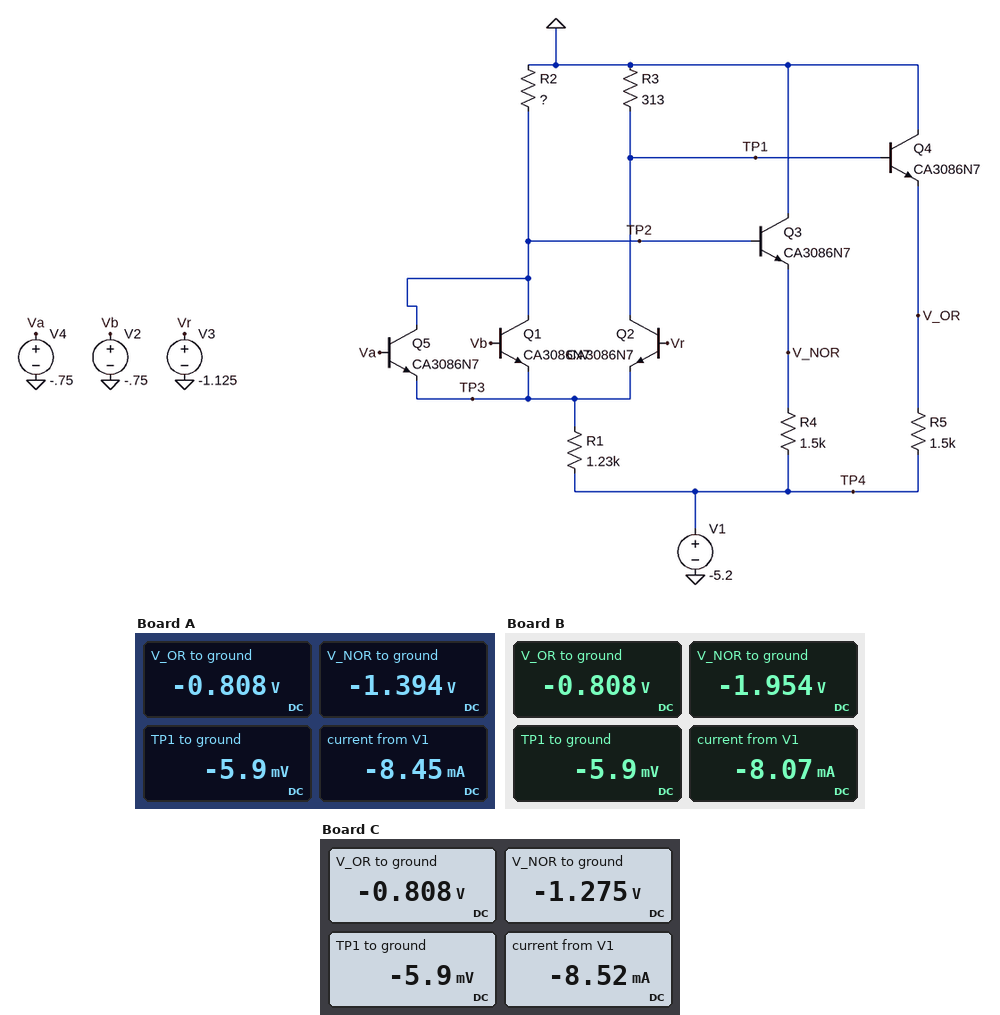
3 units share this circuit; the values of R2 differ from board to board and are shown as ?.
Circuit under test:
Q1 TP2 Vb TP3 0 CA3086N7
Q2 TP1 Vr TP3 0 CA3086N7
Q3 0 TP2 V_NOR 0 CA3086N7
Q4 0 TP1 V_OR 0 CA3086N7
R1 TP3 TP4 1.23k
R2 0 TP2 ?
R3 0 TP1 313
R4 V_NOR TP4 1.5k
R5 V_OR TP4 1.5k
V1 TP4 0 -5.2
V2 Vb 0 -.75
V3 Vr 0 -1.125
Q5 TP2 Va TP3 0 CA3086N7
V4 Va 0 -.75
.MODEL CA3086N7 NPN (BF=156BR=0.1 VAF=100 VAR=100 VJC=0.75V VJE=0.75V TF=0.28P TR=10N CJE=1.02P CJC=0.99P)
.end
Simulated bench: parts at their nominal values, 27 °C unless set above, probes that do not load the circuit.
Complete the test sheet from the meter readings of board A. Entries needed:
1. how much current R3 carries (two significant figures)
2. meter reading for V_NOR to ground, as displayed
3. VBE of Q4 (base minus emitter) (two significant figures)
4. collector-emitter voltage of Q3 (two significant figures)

19 µA
-1.394 V
800 mV
1.4 V
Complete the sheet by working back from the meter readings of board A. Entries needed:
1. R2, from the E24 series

200 Ω
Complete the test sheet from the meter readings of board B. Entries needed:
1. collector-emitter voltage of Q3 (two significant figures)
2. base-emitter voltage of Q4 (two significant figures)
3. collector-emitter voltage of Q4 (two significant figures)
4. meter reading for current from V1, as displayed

2.0 V
800 mV
810 mV
-8.07 mA
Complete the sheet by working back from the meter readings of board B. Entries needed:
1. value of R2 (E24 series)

390 Ω
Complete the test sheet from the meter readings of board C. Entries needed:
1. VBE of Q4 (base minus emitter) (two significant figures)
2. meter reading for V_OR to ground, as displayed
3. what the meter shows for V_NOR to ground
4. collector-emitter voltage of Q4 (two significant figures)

800 mV
-0.808 V
-1.275 V
810 mV
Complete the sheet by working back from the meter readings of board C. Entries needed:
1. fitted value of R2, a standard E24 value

160 Ω
